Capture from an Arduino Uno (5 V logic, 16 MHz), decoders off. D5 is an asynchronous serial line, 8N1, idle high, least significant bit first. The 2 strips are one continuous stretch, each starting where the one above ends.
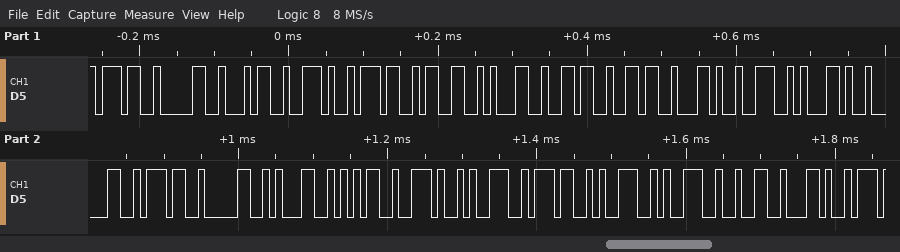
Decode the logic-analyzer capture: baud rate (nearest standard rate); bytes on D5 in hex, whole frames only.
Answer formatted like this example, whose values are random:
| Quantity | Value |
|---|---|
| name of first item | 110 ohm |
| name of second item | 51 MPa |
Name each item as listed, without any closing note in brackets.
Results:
| Quantity | Value |
|---|---|
| baud rate | 115200 baud |
| bytes on D5 in hex, whole frames only | 37 30 34 2E 37 33 31 36 36 2C 4E 2C 30 37 30 31 35 2E 39 37 39 39 32 2C |
